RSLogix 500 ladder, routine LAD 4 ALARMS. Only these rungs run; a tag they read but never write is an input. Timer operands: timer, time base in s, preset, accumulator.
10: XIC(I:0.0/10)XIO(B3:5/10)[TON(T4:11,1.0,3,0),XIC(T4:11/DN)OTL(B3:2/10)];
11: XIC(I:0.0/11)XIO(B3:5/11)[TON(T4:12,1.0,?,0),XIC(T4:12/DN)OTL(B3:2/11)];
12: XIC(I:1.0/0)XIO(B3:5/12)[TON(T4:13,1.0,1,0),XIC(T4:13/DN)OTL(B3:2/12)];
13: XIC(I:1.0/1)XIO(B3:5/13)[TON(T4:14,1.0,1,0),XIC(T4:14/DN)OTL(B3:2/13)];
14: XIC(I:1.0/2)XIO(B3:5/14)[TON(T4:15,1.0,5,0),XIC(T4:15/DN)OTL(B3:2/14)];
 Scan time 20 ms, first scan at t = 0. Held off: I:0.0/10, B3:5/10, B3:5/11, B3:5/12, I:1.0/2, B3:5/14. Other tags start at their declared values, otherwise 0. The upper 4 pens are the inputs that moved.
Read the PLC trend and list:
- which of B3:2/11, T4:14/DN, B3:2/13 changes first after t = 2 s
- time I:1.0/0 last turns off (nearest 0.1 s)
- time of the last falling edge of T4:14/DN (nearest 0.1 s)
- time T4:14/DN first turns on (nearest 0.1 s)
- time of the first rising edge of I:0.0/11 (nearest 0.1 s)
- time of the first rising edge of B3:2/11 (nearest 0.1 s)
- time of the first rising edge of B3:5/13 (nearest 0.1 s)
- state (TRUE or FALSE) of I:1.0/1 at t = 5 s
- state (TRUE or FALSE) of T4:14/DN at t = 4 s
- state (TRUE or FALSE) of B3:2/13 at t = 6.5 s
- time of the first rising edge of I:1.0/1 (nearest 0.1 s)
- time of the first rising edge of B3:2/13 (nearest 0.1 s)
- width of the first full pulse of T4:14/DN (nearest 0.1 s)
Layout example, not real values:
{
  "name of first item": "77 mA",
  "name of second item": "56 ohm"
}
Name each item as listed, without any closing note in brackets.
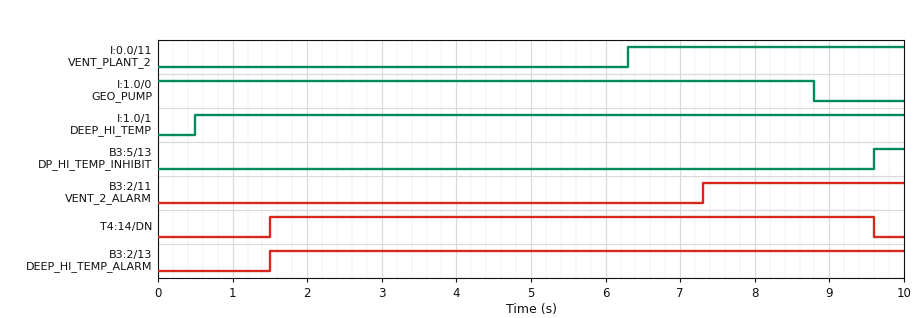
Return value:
{
  "which of B3:2/11, T4:14/DN, B3:2/13 changes first after t = 2 s": "B3:2/11",
  "time I:1.0/0 last turns off": "8.8 s",
  "time of the last falling edge of T4:14/DN": "9.6 s",
  "time T4:14/DN first turns on": "1.5 s",
  "time of the first rising edge of I:0.0/11": "6.3 s",
  "time of the first rising edge of B3:2/11": "7.3 s",
  "time of the first rising edge of B3:5/13": "9.6 s",
  "state (TRUE or FALSE) of I:1.0/1 at t = 5 s": "TRUE",
  "state (TRUE or FALSE) of T4:14/DN at t = 4 s": "TRUE",
  "state (TRUE or FALSE) of B3:2/13 at t = 6.5 s": "TRUE",
  "time of the first rising edge of I:1.0/1": "0.5 s",
  "time of the first rising edge of B3:2/13": "1.5 s",
  "width of the first full pulse of T4:14/DN": "8.1 s"
}
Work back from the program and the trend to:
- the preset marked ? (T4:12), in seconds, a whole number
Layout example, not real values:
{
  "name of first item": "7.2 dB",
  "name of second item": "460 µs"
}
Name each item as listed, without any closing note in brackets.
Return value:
{
  "the preset marked ? (T4:12), in seconds, a whole number": "1 s"
}
